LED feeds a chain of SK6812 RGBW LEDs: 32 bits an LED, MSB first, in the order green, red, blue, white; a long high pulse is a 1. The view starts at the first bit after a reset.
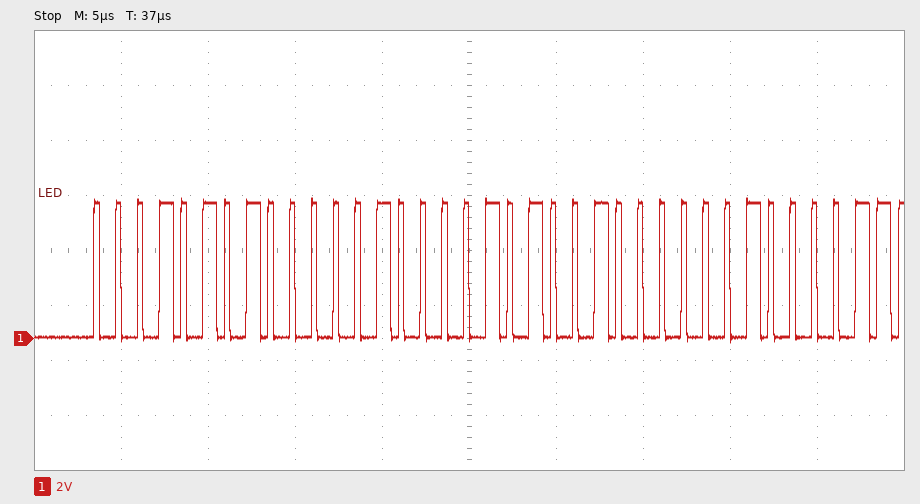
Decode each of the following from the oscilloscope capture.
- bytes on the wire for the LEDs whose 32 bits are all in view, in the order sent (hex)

15 04 29 02
